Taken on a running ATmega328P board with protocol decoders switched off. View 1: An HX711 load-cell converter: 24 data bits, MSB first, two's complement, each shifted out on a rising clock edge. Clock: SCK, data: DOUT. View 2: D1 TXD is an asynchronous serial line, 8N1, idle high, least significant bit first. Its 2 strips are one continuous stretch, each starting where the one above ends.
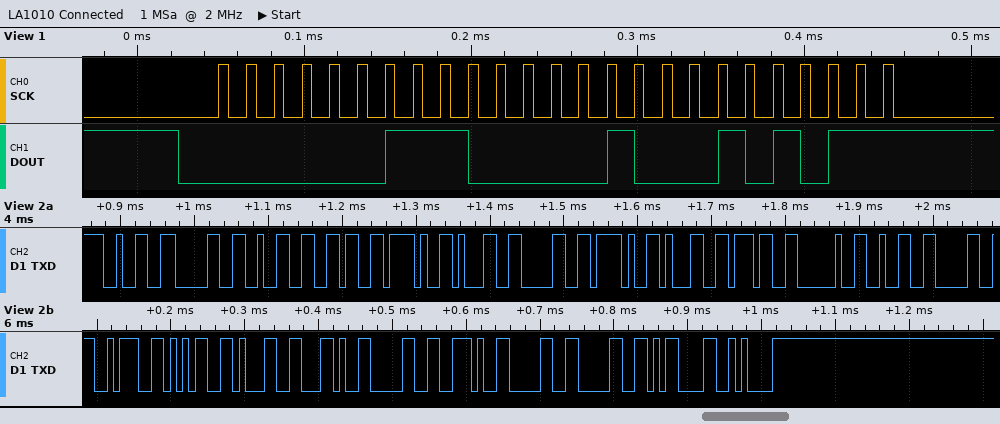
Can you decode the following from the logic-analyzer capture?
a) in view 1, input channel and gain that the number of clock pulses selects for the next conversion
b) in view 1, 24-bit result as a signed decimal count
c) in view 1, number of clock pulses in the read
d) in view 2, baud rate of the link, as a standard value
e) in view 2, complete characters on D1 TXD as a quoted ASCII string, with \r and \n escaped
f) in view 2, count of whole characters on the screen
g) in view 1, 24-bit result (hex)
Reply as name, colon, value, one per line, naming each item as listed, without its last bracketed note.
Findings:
in view 1, input channel and gain that the number of clock pulses selects for the next conversion: channel A, gain 128
in view 1, 24-bit result as a signed decimal count: 229931
in view 1, number of clock pulses in the read: 25
in view 2, baud rate of the link, as a standard value: 115200 baud
in view 2, complete characters on D1 TXD as a quoted ASCII string, with \r and \n escaped: "2026/10/17 20:51,0.00\r\n"
in view 2, count of whole characters on the screen: 23
in view 1, 24-bit result: 0x03822B
